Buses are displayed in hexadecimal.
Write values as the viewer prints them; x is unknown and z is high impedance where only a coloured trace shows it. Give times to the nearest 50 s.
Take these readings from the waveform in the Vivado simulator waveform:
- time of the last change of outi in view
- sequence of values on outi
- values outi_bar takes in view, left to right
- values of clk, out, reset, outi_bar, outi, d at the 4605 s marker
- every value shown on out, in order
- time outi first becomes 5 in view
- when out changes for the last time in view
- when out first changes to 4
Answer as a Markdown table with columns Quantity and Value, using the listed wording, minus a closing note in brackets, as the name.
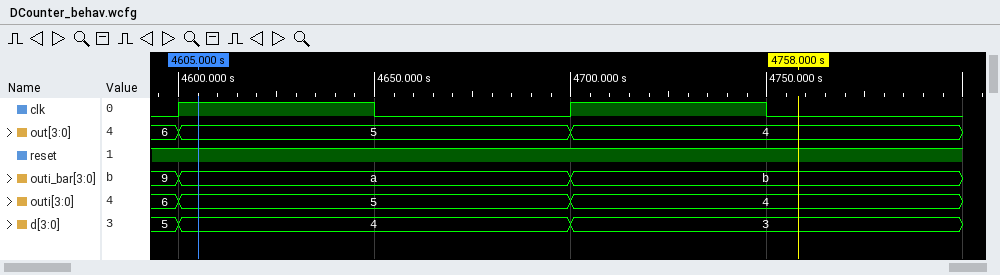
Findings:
| Quantity | Value |
|---|---|
| time of the last change of outi in view | 4700 s |
| sequence of values on outi | 6, 5, 4 |
| values outi_bar takes in view, left to right | 9, a, b |
| values of clk, out, reset, outi_bar, outi, d at the 4605 s marker | clk=1, out=5, reset=1, outi_bar=a, outi=5, d=4 |
| every value shown on out, in order | 6, 5, 4 |
| time outi first becomes 5 in view | 4600 s |
| when out changes for the last time in view | 4700 s |
| when out first changes to 4 | 4700 s |
